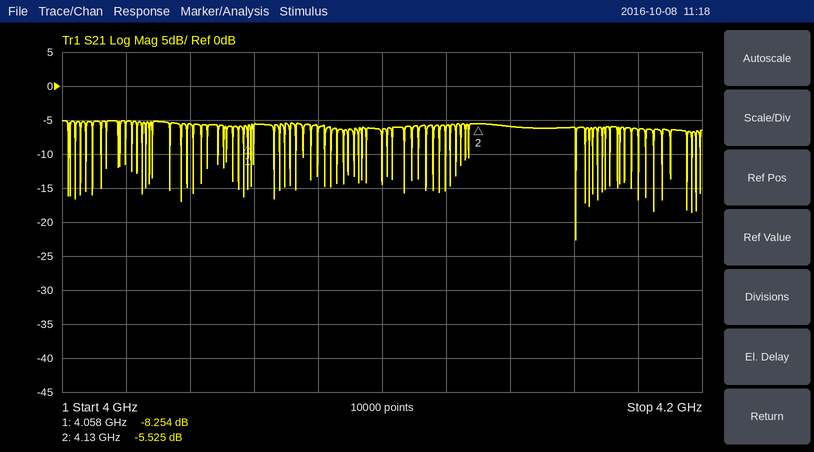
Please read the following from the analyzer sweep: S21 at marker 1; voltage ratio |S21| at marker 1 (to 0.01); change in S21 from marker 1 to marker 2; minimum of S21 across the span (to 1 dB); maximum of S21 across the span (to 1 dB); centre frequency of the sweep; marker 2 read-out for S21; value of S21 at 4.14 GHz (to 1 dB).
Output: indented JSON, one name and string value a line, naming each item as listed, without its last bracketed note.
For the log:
{
  "S21 at marker 1": "-8.254 dB",
  "voltage ratio |S21| at marker 1": "0.39",
  "change in S21 from marker 1 to marker 2": "2.729 dB",
  "minimum of S21 across the span": "-23 dB",
  "maximum of S21 across the span": "-5 dB",
  "centre frequency of the sweep": "4.1 GHz",
  "marker 2 read-out for S21": "-5.525 dB",
  "value of S21 at 4.14 GHz": "-6 dB"
}
